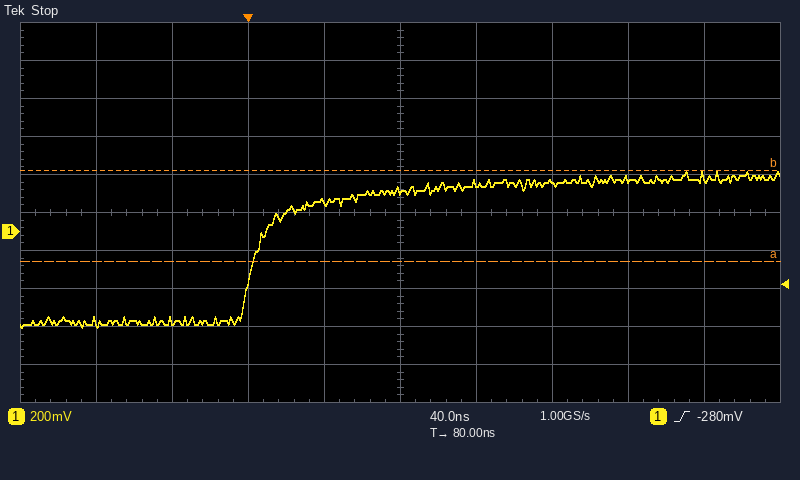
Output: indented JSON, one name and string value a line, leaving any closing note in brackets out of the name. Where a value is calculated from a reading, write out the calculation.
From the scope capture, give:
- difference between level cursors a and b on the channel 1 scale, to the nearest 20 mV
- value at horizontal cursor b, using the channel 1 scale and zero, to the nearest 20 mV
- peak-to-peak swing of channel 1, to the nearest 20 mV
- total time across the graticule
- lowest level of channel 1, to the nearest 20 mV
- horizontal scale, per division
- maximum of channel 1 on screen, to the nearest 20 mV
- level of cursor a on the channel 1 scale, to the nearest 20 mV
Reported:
{
  "difference between level cursors a and b on the channel 1 scale, to the nearest 20 mV": "480 mV",
  "value at horizontal cursor b, using the channel 1 scale and zero, to the nearest 20 mV": "320 mV",
  "peak-to-peak swing of channel 1, to the nearest 20 mV": "320 mV − (-500 mV) = 820 mV",
  "total time across the graticule": "400 ns",
  "lowest level of channel 1, to the nearest 20 mV": "-500 mV",
  "horizontal scale, per division": "40 ns",
  "maximum of channel 1 on screen, to the nearest 20 mV": "320 mV",
  "level of cursor a on the channel 1 scale, to the nearest 20 mV": "-160 mV"
}
